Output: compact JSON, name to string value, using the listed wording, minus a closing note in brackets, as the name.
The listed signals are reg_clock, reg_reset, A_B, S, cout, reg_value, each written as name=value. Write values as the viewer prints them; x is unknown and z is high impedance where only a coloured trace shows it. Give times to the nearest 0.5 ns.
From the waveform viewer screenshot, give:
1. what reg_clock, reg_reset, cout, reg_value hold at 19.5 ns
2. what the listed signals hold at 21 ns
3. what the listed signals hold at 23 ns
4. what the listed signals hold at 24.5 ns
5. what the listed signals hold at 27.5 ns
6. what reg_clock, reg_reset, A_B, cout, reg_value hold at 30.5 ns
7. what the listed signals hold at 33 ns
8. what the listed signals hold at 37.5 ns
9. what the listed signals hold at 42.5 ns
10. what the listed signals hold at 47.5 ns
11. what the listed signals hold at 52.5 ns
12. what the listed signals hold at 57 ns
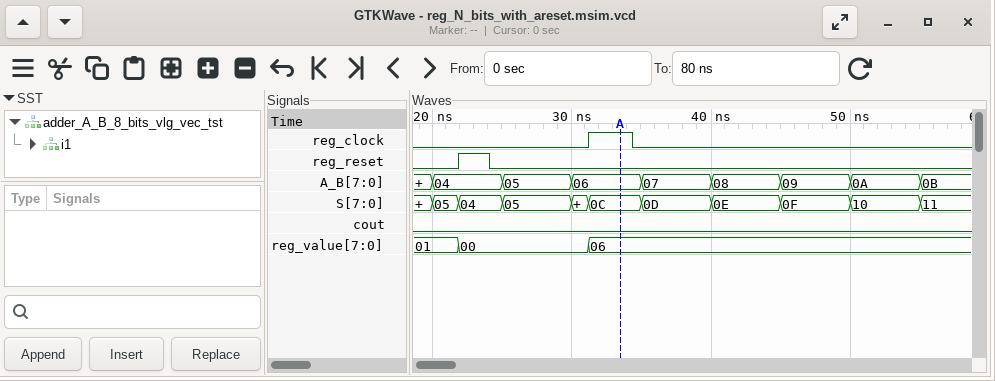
{"what reg_clock, reg_reset, cout, reg_value hold at 19.5 ns": "reg_clock=0, reg_reset=0, cout=0, reg_value=01", "what the listed signals hold at 21 ns": "reg_clock=0, reg_reset=0, A_B=04, S=05, cout=0, reg_value=01", "what the listed signals hold at 23 ns": "reg_clock=0, reg_reset=1, A_B=04, S=04, cout=0, reg_value=00", "what the listed signals hold at 24.5 ns": "reg_clock=0, reg_reset=0, A_B=04, S=04, cout=0, reg_value=00", "what the listed signals hold at 27.5 ns": "reg_clock=0, reg_reset=0, A_B=05, S=05, cout=0, reg_value=00", "what reg_clock, reg_reset, A_B, cout, reg_value hold at 30.5 ns": "reg_clock=0, reg_reset=0, A_B=06, cout=0, reg_value=00", "what the listed signals hold at 33 ns": "reg_clock=1, reg_reset=0, A_B=06, S=0C, cout=0, reg_value=06", "what the listed signals hold at 37.5 ns": "reg_clock=0, reg_reset=0, A_B=07, S=0D, cout=0, reg_value=06", "what the listed signals hold at 42.5 ns": "reg_clock=0, reg_reset=0, A_B=08, S=0E, cout=0, reg_value=06", "what the listed signals hold at 47.5 ns": "reg_clock=0, reg_reset=0, A_B=09, S=0F, cout=0, reg_value=06", "what the listed signals hold at 52.5 ns": "reg_clock=0, reg_reset=0, A_B=0A, S=10, cout=0, reg_value=06", "what the listed signals hold at 57 ns": "reg_clock=0, reg_reset=0, A_B=0B, S=11, cout=0, reg_value=06"}
